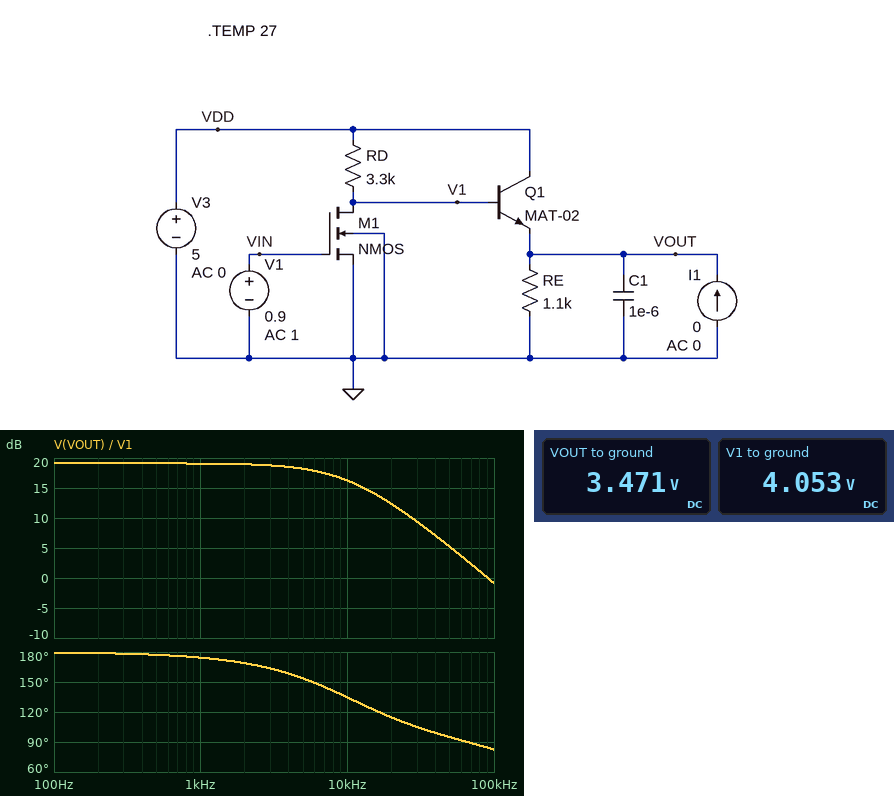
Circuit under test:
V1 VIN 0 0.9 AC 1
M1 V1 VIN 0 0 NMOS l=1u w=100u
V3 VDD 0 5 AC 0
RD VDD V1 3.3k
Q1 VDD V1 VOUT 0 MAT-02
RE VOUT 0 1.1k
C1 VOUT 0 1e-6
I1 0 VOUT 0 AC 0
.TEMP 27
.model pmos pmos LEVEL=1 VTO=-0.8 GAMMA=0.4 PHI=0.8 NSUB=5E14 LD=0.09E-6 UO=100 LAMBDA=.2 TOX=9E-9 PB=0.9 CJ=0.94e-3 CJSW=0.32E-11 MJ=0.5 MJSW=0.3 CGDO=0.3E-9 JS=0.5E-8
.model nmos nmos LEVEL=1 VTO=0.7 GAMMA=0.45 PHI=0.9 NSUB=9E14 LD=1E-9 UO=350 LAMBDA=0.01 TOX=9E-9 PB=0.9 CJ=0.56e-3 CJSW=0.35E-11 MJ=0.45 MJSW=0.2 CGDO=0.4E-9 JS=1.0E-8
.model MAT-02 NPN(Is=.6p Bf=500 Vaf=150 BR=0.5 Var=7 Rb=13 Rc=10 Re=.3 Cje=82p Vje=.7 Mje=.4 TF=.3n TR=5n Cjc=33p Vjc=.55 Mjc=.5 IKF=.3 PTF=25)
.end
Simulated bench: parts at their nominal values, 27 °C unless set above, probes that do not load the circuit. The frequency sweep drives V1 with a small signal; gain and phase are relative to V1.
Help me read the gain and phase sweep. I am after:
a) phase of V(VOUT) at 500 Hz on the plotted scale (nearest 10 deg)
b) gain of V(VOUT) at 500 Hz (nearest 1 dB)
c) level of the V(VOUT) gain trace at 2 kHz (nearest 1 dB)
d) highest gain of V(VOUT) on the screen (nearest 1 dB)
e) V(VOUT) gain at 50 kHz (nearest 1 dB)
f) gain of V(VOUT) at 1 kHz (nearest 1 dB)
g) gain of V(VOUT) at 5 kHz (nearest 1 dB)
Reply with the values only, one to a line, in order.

180 deg
19 dB
19 dB
19 dB
5 dB
19 dB
18 dB
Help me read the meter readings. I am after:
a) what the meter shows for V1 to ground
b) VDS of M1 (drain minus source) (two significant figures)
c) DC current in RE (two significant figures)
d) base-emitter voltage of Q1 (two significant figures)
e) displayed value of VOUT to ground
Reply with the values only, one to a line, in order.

4.053 V
4.1 V
3.2 mA
580 mV
3.471 V
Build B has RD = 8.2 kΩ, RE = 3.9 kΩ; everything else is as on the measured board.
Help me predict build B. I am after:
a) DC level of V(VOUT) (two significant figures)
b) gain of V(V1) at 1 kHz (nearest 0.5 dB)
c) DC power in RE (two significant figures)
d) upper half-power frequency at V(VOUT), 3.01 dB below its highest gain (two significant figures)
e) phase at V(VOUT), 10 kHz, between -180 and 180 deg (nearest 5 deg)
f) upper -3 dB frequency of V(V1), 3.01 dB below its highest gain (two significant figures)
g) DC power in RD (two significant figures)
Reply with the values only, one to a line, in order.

2.2 V
26.5 dB
1.2 mW
2.6 kHz
100 deg
57 kHz
630 µW
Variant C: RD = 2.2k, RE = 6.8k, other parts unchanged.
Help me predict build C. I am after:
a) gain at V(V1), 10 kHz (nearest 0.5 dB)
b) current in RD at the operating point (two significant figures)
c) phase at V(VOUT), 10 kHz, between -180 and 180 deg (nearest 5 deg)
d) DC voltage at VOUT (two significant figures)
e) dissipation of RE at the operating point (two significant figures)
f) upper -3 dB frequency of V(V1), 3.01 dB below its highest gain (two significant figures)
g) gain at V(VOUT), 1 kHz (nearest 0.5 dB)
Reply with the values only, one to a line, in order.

15.0 dB
280 µA
105 deg
3.8 V
2.2 mW
390 kHz
15.5 dB
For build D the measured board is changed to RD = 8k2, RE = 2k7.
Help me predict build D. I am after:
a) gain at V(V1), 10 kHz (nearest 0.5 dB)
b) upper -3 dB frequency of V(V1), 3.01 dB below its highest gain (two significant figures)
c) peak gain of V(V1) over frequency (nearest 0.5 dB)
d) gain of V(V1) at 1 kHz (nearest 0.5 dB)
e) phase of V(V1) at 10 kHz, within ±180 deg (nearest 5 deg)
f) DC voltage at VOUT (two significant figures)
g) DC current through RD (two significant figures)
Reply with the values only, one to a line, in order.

24.0 dB
10 kHz
27.0 dB
26.5 dB
170 deg
2.2 V
280 µA
